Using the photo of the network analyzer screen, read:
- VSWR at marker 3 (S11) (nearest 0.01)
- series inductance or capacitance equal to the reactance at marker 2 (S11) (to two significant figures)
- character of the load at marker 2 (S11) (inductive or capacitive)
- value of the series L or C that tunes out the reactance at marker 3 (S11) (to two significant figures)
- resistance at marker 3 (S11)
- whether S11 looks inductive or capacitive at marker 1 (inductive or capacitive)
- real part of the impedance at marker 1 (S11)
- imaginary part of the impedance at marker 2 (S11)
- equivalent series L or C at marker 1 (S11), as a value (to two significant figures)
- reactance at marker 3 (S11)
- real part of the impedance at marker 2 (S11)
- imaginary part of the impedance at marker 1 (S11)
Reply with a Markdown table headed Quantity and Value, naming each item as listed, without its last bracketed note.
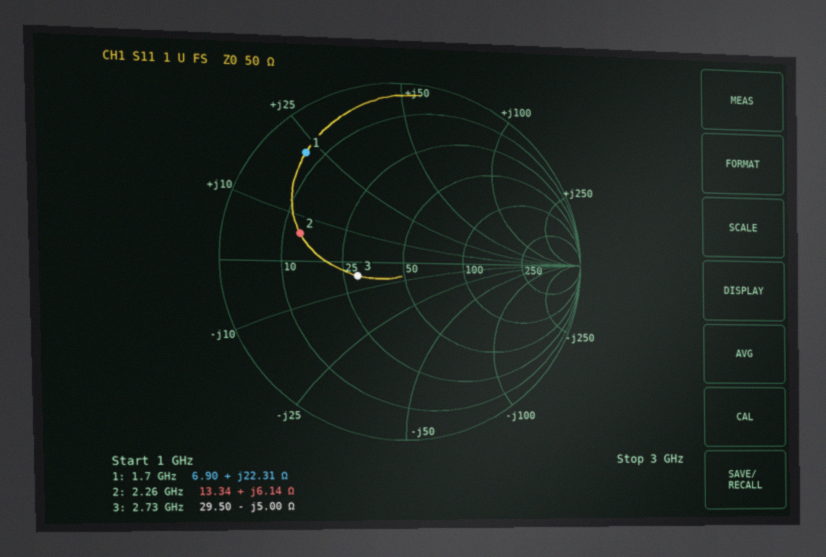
| Quantity | Value |
|---|---|
| VSWR at marker 3 (S11) | 1.72 |
| series inductance or capacitance equal to the reactance at marker 2 (S11) | 430 pH |
| character of the load at marker 2 (S11) | inductive |
| value of the series L or C that tunes out the reactance at marker 3 (S11) | 290 pH |
| resistance at marker 3 | 29.50 Ω |
| whether S11 looks inductive or capacitive at marker 1 | inductive |
| real part of the impedance at marker 1 | 6.90 Ω |
| imaginary part of the impedance at marker 2 | +6.14 Ω |
| equivalent series L or C at marker 1 (S11), as a value | 2.1 nH |
| reactance at marker 3 | -5.00 Ω |
| real part of the impedance at marker 2 | 13.34 Ω |
| imaginary part of the impedance at marker 1 | +22.31 Ω |
